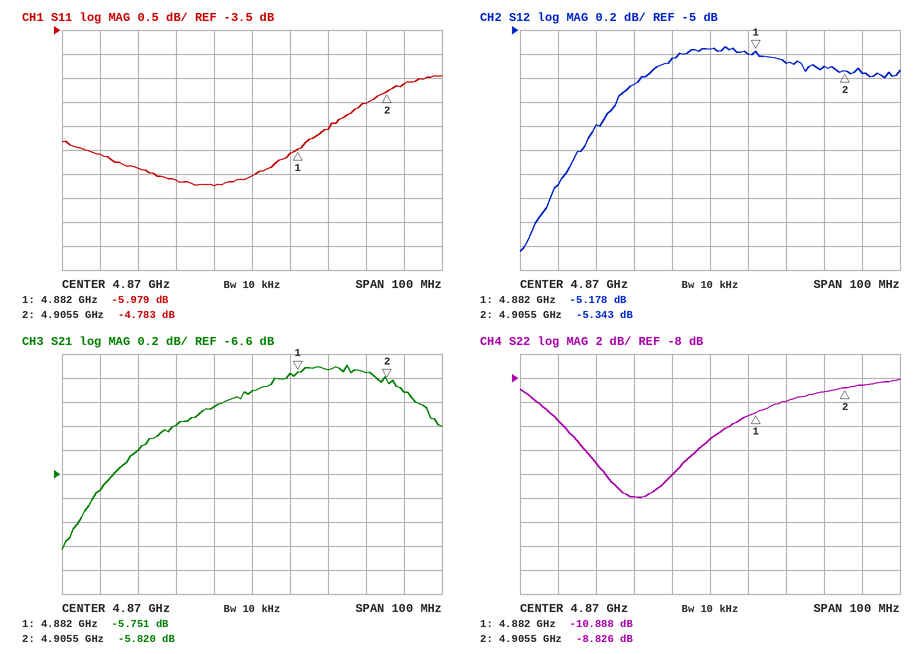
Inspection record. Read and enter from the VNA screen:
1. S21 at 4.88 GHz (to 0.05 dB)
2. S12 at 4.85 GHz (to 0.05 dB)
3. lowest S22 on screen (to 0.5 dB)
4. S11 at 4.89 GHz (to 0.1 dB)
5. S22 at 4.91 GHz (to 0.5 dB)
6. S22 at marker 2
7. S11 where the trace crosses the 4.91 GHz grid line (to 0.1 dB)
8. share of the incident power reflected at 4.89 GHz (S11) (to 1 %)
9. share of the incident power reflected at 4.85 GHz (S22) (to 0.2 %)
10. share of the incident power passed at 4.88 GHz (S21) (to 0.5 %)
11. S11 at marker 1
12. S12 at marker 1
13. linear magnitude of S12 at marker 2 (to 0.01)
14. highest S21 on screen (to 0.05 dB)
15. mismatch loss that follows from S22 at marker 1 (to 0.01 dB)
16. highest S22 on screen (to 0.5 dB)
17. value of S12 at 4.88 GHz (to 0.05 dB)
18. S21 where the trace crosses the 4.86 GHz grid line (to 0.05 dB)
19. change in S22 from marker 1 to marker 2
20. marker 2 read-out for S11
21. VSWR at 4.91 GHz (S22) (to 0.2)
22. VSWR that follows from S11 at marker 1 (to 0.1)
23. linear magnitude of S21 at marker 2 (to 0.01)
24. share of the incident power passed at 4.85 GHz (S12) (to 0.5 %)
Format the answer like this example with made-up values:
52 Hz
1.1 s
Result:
-5.75 dB
-5.45 dB
-18.0 dB
-5.6 dB
-8.5 dB
-8.826 dB
-4.6 dB
28 %
1.6 %
26.5 %
-5.979 dB
-5.178 dB
0.54
-5.70 dB
0.37 dB
-8.0 dB
-5.20 dB
-6.05 dB
2.062 dB
-4.783 dB
2.2
3.0
0.51
28.5 %
